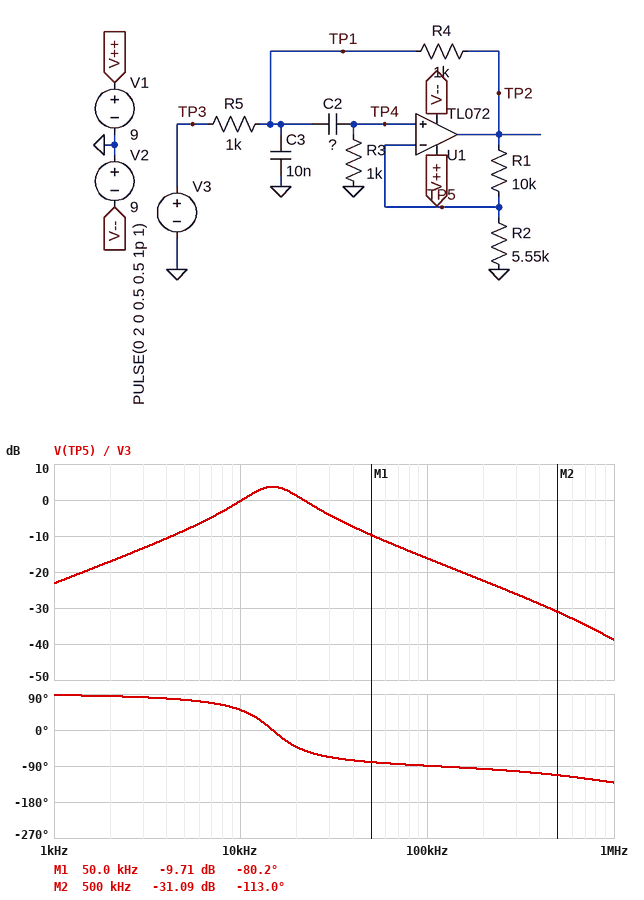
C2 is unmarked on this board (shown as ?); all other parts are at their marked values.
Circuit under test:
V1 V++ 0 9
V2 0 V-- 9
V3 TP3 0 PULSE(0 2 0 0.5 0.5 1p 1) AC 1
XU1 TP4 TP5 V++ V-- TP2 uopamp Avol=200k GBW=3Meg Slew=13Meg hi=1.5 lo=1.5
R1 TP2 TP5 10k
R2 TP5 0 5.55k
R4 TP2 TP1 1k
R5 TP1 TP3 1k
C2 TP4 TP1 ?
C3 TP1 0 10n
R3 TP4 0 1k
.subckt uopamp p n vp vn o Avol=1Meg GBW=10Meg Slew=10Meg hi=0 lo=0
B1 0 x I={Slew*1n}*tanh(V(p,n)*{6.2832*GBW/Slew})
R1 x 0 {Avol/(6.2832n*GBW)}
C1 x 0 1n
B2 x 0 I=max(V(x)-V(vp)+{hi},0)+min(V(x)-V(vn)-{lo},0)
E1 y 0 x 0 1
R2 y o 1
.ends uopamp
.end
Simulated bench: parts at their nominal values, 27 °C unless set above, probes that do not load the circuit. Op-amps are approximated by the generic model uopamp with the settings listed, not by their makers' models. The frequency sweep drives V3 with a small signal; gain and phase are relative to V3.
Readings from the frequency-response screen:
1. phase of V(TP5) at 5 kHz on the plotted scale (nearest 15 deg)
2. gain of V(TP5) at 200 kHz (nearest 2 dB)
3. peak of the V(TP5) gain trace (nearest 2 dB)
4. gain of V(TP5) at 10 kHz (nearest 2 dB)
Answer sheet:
75 deg
-22 dB
4 dB
0 dB
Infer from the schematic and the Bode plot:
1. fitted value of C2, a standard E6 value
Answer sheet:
22 nF
